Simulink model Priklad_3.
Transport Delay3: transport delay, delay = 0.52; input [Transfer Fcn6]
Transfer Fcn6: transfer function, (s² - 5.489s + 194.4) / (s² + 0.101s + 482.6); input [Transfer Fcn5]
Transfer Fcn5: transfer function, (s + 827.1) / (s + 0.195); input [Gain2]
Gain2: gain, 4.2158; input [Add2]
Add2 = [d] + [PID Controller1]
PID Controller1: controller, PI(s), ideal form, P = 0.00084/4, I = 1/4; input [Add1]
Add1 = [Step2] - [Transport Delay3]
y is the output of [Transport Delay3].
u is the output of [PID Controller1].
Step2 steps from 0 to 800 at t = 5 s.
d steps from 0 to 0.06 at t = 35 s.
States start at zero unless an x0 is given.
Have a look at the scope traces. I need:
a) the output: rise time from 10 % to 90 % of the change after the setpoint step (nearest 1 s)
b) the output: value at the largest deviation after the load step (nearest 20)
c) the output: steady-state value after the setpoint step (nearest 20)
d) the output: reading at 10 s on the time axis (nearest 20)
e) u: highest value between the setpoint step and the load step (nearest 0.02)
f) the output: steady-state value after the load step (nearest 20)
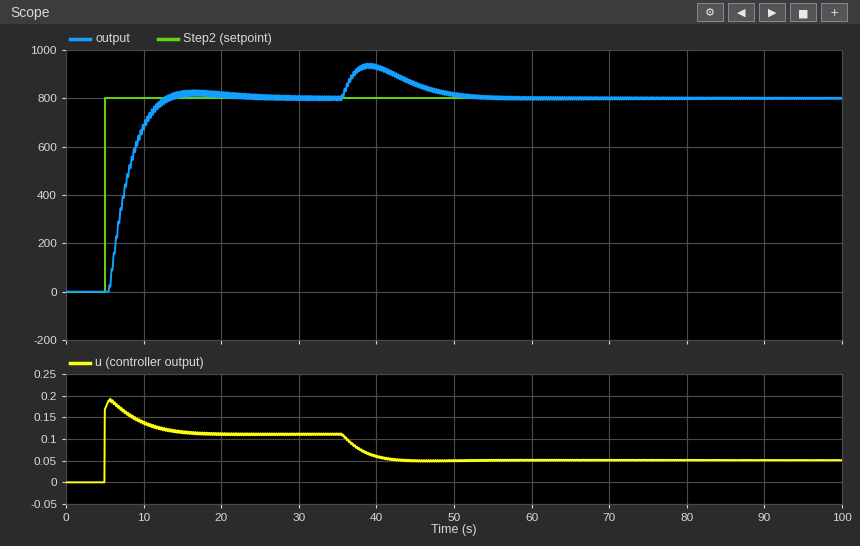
5 s
940
800
680
0.20
800
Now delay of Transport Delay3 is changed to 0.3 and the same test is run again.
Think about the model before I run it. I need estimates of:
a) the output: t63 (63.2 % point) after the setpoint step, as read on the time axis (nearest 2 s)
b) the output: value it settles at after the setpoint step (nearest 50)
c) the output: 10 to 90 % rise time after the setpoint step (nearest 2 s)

8 s
800
6 s
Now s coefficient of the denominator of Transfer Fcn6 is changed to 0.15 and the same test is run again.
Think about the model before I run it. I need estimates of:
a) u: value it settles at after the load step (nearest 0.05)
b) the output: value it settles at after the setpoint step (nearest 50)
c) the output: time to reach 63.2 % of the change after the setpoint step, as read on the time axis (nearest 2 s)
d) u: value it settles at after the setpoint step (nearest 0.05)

0.05
800
8 s
0.10
